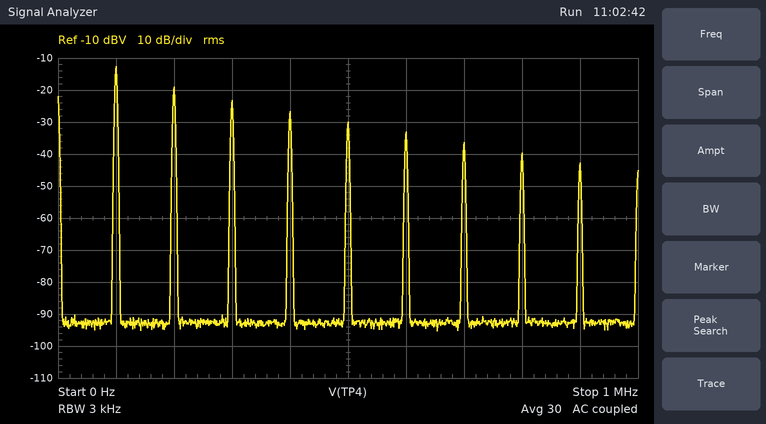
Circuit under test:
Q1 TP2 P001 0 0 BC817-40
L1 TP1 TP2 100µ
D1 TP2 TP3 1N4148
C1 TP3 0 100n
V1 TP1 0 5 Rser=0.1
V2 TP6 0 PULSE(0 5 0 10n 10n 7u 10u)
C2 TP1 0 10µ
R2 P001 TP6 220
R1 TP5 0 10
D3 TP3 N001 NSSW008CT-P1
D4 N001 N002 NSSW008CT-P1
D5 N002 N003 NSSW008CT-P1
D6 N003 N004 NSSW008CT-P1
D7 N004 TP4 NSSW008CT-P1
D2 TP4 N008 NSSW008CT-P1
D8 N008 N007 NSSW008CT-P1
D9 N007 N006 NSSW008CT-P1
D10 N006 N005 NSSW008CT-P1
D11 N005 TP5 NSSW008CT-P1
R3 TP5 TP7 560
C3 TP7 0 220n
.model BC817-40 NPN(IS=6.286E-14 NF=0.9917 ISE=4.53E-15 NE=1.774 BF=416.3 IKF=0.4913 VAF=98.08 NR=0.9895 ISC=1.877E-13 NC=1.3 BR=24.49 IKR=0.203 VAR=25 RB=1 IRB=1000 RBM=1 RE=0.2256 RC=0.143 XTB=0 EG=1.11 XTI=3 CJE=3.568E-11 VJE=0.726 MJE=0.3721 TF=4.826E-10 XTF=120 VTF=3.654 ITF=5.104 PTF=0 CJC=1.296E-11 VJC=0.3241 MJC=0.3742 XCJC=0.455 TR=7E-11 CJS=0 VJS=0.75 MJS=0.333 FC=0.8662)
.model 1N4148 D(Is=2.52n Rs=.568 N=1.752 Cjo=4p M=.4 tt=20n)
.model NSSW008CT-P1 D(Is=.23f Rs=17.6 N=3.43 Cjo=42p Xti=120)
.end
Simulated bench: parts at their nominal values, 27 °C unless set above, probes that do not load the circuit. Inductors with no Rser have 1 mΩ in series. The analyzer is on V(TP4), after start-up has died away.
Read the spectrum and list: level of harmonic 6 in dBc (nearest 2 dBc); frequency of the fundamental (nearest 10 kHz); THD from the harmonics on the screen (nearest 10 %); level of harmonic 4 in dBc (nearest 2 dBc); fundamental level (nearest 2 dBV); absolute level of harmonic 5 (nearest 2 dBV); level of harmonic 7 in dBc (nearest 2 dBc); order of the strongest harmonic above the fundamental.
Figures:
-20 dBc
100 kHz
60 %
-14 dBc
-12 dBV
-30 dBV
-24 dBc
2
